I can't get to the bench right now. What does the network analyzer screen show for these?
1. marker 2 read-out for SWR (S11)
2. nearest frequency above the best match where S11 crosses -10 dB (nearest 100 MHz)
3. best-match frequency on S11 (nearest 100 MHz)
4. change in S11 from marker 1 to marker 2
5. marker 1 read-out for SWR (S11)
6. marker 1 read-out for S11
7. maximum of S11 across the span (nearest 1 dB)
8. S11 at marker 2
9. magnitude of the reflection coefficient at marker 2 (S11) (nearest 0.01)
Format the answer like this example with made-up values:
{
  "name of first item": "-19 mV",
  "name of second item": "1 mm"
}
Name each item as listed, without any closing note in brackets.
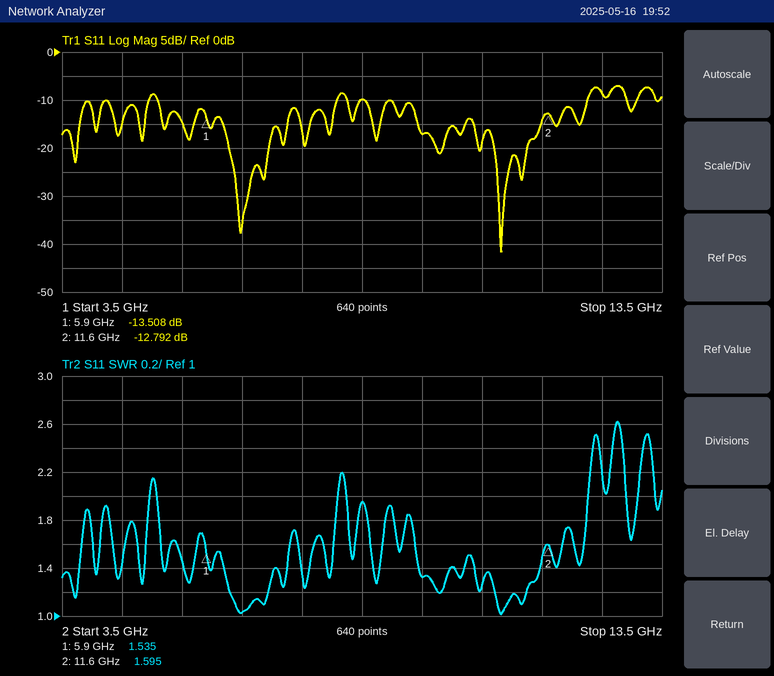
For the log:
{
  "marker 2 read-out for SWR": "1.595",
  "nearest frequency above the best match where S11 crosses -10 dB": "12.3 GHz",
  "best-match frequency on S11": "10.8 GHz",
  "change in S11 from marker 1 to marker 2": "0.716 dB",
  "marker 1 read-out for SWR": "1.535",
  "marker 1 read-out for S11": "-13.508 dB",
  "maximum of S11 across the span": "-7 dB",
  "S11 at marker 2": "-12.792 dB",
  "magnitude of the reflection coefficient at marker 2 (S11)": "0.23"
}
